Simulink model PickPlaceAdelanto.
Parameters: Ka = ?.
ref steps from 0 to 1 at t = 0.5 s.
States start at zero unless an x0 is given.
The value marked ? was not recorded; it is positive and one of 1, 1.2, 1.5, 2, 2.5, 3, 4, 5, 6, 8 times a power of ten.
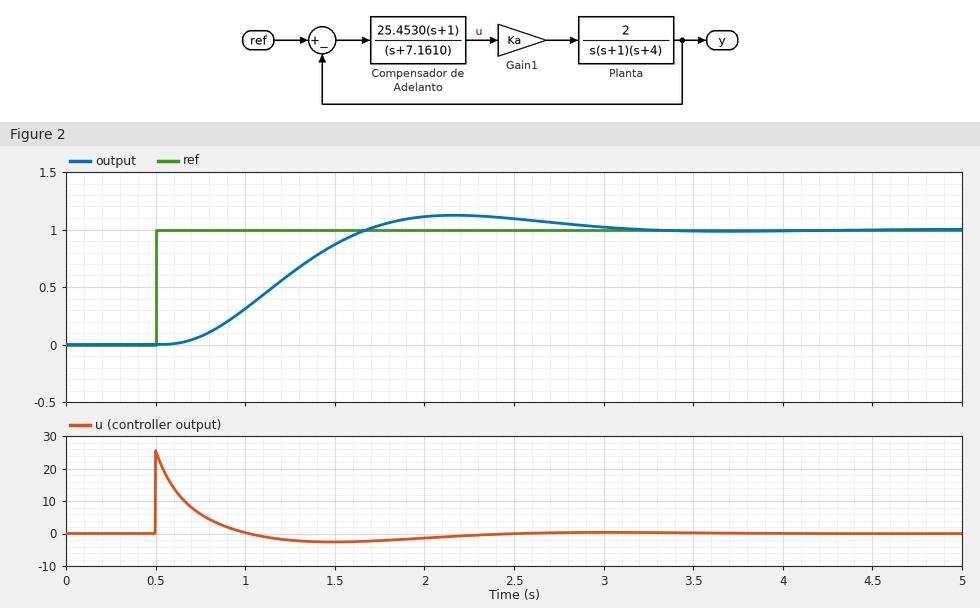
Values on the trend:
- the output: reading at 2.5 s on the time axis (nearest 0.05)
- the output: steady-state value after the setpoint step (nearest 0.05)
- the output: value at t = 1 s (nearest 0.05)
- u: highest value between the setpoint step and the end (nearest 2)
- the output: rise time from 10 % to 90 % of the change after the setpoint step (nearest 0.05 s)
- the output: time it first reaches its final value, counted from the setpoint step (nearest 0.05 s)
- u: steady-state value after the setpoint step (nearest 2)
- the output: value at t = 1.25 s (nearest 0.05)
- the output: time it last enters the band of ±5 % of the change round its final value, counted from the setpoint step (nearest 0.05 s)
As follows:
1.10
1.00
0.30
26
0.75 s
1.20 s
0
0.60
2.30 s
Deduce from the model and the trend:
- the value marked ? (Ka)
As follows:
1
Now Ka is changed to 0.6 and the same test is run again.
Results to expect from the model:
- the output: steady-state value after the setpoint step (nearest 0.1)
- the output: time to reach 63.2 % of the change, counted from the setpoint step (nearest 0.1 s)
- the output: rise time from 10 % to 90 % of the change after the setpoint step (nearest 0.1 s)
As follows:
1.0
1.1 s
1.3 s
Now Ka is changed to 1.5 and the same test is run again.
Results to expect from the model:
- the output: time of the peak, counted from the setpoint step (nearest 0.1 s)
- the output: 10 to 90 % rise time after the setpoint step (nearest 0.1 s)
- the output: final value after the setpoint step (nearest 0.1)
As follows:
1.3 s
0.5 s
1.0
